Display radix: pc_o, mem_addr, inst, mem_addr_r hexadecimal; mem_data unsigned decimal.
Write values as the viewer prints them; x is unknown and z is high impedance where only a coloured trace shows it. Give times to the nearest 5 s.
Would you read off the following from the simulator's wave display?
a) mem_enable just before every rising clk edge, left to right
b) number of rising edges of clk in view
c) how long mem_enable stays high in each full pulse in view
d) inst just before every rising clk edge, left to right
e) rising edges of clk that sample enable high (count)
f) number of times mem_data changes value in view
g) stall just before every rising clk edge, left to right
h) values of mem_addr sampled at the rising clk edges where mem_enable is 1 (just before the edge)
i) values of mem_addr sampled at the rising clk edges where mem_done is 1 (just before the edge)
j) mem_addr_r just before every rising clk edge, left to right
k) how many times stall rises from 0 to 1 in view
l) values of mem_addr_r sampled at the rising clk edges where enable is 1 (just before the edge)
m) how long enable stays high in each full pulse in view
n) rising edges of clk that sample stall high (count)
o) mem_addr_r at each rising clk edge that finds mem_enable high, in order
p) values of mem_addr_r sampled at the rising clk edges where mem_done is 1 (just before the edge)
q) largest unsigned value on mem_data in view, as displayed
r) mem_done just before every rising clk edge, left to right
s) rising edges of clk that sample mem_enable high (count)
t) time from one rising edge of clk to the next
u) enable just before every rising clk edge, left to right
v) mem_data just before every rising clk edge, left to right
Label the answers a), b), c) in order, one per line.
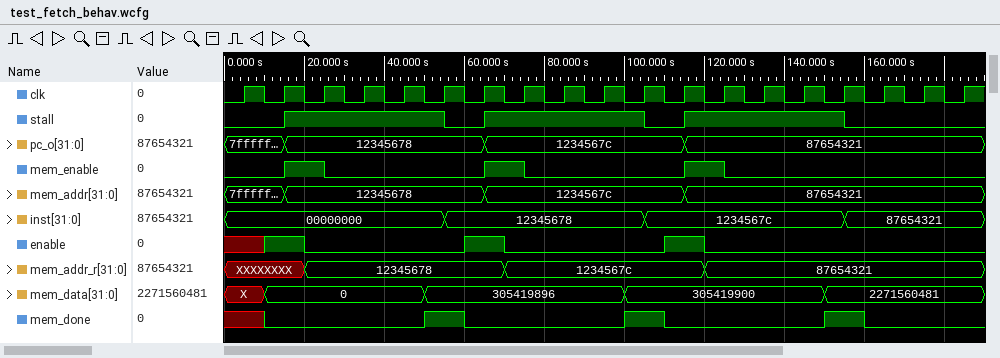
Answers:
a) 0 0 1 0 0 0 0 1 0 0 0 0 1 0 0 0 0 0 0
b) 19
c) 10 s, 10 s, 10 s
d) 00000000, 00000000, 00000000, 00000000, 00000000, 00000000, 12345678, 12345678, 12345678, 12345678, 12345678, 1234567c, 1234567c, 1234567c, 1234567c, 1234567c, 87654321, 87654321, 87654321
e) 3
f) 4
g) 0 0 1 1 1 1 0 1 1 1 1 0 1 1 1 1 0 0 0
h) 12345678, 1234567c, 87654321
i) 12345678, 1234567c, 87654321
j) XXXXXXXX, XXXXXXXX, 12345678, 12345678, 12345678, 12345678, 12345678, 1234567c, 1234567c, 1234567c, 1234567c, 1234567c, 87654321, 87654321, 87654321, 87654321, 87654321, 87654321, 87654321
k) 3
l) XXXXXXXX, 12345678, 1234567c
m) 10 s, 10 s
n) 12
o) 12345678, 1234567c, 87654321
p) 12345678, 1234567c, 87654321
q) 2271560481
r) x 0 0 0 0 1 0 0 0 0 1 0 0 0 0 1 0 0 0
s) 3
t) 10 s
u) x 1 0 0 0 0 1 0 0 0 0 1 0 0 0 0 0 0 0
v) X, 0, 0, 0, 0, 305419896, 305419896, 305419896, 305419896, 305419896, 305419900, 305419900, 305419900, 305419900, 305419900, 2271560481, 2271560481, 2271560481, 2271560481
